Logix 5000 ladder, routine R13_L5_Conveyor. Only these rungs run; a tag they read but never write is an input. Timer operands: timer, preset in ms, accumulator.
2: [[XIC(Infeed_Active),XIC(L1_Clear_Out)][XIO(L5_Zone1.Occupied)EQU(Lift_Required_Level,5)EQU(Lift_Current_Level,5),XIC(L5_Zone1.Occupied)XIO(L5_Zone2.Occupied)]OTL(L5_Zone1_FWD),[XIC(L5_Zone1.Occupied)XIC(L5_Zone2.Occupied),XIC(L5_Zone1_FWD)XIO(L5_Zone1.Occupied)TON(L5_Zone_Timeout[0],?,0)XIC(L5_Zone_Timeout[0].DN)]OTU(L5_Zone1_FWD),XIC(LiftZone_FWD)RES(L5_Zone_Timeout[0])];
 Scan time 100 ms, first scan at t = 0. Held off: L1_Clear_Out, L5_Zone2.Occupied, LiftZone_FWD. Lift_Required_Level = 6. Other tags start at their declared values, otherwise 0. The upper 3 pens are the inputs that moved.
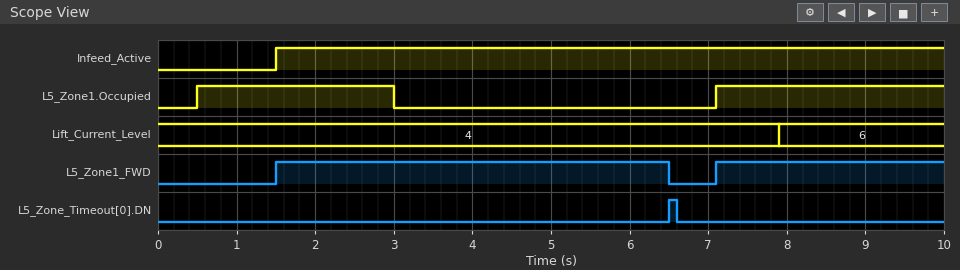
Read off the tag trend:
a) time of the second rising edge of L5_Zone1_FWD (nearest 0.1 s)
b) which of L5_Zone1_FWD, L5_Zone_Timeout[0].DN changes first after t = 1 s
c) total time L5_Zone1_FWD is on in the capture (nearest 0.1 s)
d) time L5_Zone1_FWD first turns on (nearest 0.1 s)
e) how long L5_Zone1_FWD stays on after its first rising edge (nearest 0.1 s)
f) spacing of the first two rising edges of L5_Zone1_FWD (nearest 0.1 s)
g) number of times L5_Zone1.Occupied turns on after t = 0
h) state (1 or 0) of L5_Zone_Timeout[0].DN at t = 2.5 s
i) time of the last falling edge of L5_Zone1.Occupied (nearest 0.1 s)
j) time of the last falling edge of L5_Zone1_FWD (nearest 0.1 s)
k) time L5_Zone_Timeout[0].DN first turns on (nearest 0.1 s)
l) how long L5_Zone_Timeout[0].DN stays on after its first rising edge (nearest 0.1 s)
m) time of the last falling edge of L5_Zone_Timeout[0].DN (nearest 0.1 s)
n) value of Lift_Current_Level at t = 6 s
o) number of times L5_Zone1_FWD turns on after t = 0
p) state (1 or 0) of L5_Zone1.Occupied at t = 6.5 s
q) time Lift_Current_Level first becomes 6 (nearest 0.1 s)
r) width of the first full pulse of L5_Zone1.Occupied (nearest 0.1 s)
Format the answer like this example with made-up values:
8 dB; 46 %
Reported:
7.1 s; L5_Zone1_FWD; 7.9 s; 1.5 s; 5.0 s; 5.6 s; 2; 0; 3.0 s; 6.5 s; 6.5 s; 0.1 s; 6.6 s; 4; 2; 0; 7.9 s; 2.5 s
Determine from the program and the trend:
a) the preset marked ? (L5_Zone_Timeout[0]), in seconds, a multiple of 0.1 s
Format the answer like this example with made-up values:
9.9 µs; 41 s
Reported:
3.5 s
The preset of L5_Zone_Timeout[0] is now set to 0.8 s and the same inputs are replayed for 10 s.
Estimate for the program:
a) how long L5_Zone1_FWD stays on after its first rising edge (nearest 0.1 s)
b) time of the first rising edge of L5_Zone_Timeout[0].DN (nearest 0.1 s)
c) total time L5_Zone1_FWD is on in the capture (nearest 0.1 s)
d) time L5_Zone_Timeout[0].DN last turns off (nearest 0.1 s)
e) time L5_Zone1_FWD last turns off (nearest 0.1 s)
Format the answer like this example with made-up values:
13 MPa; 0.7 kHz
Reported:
2.3 s; 3.8 s; 5.2 s; 3.9 s; 3.8 s
